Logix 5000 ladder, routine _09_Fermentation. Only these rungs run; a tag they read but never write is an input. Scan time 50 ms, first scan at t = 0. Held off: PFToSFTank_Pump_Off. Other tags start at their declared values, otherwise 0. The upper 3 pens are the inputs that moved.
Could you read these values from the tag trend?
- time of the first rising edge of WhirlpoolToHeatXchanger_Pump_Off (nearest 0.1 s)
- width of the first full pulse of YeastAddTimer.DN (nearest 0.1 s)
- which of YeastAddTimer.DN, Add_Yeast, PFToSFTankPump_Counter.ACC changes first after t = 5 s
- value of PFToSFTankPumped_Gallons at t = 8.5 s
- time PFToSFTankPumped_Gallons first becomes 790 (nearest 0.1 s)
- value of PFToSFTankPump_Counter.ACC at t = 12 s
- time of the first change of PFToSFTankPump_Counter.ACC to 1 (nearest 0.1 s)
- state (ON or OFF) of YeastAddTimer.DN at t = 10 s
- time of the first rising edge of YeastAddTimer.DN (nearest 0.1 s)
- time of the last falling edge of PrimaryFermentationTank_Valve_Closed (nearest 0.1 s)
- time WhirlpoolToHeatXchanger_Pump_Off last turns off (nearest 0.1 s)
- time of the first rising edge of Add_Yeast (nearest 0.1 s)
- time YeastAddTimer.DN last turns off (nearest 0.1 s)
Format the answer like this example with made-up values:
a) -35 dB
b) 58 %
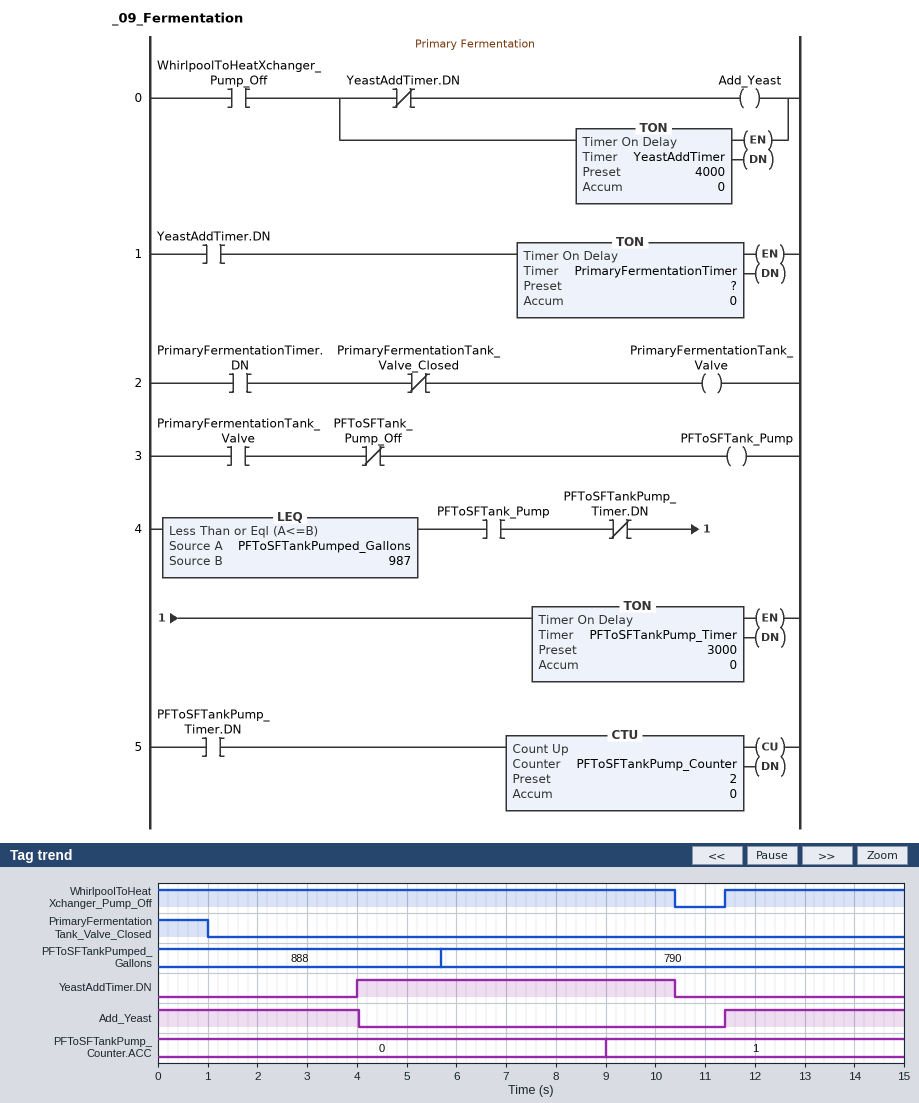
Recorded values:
a) 11.4 s
b) 6.4 s
c) PFToSFTankPump_Counter.ACC
d) 790
e) 5.7 s
f) 1
g) 9.0 s
h) ON
i) 4.0 s
j) 1.0 s
k) 10.4 s
l) 11.4 s
m) 10.4 s
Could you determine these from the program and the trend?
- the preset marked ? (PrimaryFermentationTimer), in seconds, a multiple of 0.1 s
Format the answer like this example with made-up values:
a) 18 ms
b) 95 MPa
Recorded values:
a) 2.0 s
